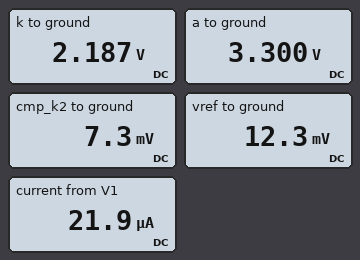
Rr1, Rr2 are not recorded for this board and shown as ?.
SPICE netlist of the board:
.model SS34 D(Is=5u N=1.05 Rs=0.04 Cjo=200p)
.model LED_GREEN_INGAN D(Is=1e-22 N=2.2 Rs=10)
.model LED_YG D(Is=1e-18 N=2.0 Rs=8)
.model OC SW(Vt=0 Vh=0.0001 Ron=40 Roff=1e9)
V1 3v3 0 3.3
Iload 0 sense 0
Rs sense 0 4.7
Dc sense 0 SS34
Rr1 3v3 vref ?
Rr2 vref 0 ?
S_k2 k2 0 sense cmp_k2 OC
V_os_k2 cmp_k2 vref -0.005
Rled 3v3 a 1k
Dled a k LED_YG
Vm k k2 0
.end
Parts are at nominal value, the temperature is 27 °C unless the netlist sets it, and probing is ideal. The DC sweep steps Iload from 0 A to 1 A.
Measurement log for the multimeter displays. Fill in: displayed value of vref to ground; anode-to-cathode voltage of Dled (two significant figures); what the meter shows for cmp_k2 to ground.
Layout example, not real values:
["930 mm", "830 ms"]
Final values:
["12.3 mV", "1.1 V", "7.3 mV"]
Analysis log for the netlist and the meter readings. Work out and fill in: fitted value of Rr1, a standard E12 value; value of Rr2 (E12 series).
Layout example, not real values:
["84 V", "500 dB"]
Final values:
["150 kΩ", "560 Ω"]
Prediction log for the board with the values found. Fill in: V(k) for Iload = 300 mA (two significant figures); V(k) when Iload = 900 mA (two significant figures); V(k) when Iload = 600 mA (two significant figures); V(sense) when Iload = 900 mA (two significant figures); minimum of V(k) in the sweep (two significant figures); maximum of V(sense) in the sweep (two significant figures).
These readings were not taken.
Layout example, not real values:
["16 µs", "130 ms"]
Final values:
["57 mV", "57 mV", "57 mV", "360 mV", "57 mV", "370 mV"]
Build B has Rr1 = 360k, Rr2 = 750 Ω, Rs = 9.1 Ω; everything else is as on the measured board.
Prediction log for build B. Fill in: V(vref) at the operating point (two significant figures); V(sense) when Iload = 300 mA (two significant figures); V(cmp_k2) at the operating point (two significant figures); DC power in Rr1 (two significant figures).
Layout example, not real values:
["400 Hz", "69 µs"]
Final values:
["6.9 mV", "310 mV", "1.9 mV", "30 µW"]
